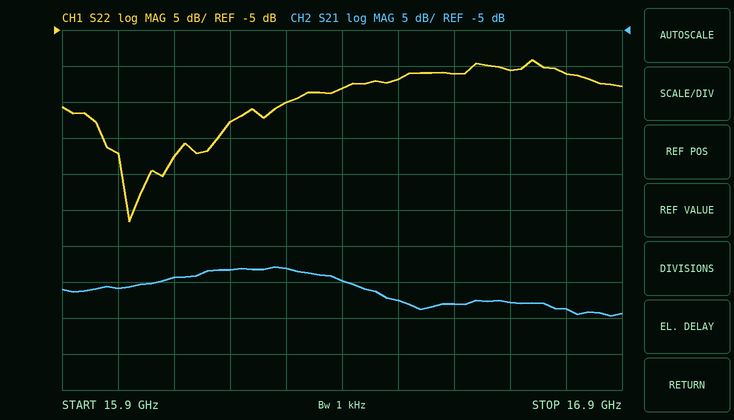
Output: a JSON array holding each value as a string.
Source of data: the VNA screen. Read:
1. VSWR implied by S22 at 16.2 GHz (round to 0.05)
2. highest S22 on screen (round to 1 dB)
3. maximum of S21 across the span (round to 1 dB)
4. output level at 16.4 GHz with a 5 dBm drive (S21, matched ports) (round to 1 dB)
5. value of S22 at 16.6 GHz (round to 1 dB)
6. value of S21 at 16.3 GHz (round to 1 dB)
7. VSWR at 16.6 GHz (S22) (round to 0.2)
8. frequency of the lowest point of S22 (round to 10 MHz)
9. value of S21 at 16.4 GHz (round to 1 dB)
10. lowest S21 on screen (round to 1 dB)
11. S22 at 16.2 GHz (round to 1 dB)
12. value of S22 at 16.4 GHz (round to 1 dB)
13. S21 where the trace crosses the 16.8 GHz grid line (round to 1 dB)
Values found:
["1.30", "-9 dB", "-38 dB", "-35 dBm", "-11 dB", "-38 dB", "1.8", "16.02 GHz", "-40 dB", "-45 dB", "-18 dB", "-13 dB", "-44 dB"]
